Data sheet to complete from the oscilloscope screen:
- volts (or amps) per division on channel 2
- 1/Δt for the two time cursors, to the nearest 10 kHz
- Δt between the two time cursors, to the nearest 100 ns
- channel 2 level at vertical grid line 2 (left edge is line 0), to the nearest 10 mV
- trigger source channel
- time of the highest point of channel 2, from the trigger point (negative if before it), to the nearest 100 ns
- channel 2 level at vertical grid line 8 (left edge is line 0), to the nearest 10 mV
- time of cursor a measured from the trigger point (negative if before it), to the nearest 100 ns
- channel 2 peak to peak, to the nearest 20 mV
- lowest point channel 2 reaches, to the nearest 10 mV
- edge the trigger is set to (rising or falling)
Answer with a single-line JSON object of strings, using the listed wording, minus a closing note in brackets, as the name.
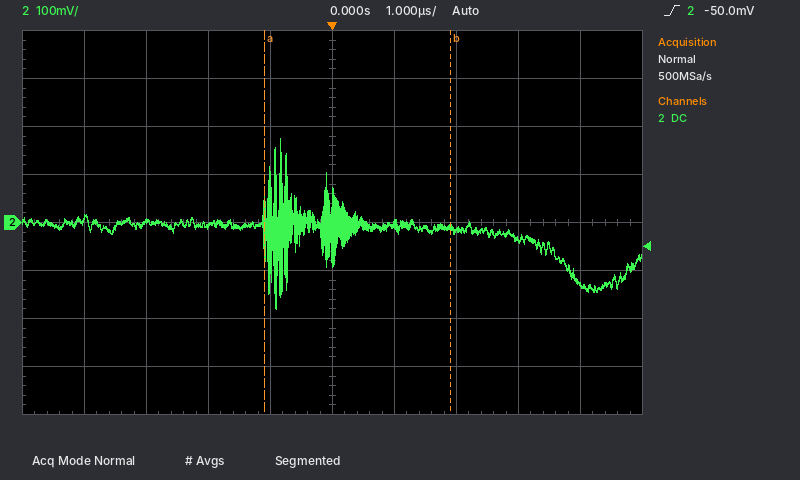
{"volts (or amps) per division on channel 2": "100 mV", "1/Δt for the two time cursors, to the nearest 10 kHz": "330 kHz", "Δt between the two time cursors, to the nearest 100 ns": "3.0 µs", "channel 2 level at vertical grid line 2 (left edge is line 0), to the nearest 10 mV": "0 mV", "trigger source channel": "channel 2", "time of the highest point of channel 2, from the trigger point (negative if before it), to the nearest 100 ns": "-800 ns", "channel 2 level at vertical grid line 8 (left edge is line 0), to the nearest 10 mV": "-40 mV", "time of cursor a measured from the trigger point (negative if before it), to the nearest 100 ns": "-1.1 µs", "channel 2 peak to peak, to the nearest 20 mV": "360 mV", "lowest point channel 2 reaches, to the nearest 10 mV": "-180 mV", "edge the trigger is set to": "rising"}
